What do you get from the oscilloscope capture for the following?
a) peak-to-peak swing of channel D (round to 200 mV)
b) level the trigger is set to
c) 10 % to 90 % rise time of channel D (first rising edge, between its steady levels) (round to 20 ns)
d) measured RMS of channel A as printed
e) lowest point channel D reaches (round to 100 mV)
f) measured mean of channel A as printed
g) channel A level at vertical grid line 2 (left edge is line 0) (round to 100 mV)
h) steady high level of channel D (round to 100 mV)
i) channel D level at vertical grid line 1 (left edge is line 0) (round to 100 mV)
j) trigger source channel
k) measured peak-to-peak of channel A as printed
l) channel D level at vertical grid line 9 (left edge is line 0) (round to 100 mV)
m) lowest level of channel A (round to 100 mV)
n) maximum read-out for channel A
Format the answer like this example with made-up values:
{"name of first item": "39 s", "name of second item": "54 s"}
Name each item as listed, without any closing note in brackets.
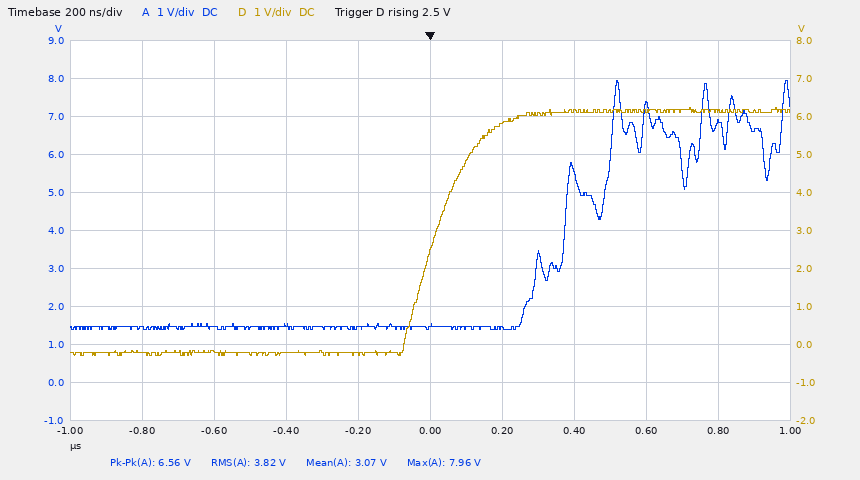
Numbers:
{"peak-to-peak swing of channel D": "6.6 V", "level the trigger is set to": "2.5 V", "10 % to 90 % rise time of channel D (first rising edge, between its steady levels)": "220 ns", "measured RMS of channel A as printed": "3.82 V", "lowest point channel D reaches": "-300 mV", "measured mean of channel A as printed": "3.07 V", "channel A level at vertical grid line 2 (left edge is line 0)": "1.5 V", "steady high level of channel D": "6.1 V", "channel D level at vertical grid line 1 (left edge is line 0)": "-200 mV", "trigger source channel": "channel D", "measured peak-to-peak of channel A as printed": "6.56 V", "channel D level at vertical grid line 9 (left edge is line 0)": "6.1 V", "lowest level of channel A": "1.4 V", "maximum read-out for channel A": "7.96 V"}
